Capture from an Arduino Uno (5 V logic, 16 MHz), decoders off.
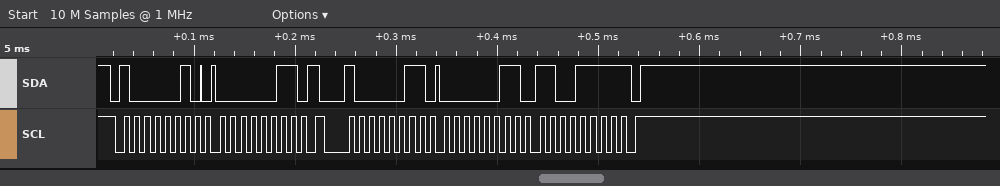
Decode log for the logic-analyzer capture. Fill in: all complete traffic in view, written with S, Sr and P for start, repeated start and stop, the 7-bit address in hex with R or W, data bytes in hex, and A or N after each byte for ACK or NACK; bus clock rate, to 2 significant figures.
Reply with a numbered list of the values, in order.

1. S 41W A 03 A Sr 41R A 03 A CF N P
2. 100 kHz
